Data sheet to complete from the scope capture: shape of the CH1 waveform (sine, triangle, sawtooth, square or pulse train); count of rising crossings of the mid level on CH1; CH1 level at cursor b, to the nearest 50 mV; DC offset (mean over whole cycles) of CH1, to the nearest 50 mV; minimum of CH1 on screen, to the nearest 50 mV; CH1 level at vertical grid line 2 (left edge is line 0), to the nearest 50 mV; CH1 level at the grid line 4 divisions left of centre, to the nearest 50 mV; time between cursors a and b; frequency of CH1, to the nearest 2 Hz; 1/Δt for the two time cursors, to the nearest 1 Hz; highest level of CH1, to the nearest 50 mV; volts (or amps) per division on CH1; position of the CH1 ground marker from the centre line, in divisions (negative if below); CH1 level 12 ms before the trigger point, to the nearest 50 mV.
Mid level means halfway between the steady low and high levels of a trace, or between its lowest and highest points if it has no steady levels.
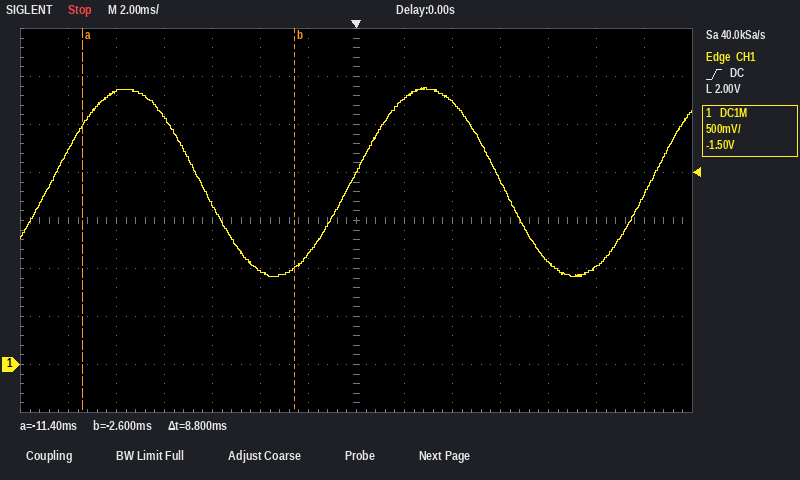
sine
3
1.00 V
1.90 V
900 mV
2.85 V
2.60 V
8.8 ms
80 Hz
114 Hz
2.90 V
500 mV
-3.0 div
2.25 V
